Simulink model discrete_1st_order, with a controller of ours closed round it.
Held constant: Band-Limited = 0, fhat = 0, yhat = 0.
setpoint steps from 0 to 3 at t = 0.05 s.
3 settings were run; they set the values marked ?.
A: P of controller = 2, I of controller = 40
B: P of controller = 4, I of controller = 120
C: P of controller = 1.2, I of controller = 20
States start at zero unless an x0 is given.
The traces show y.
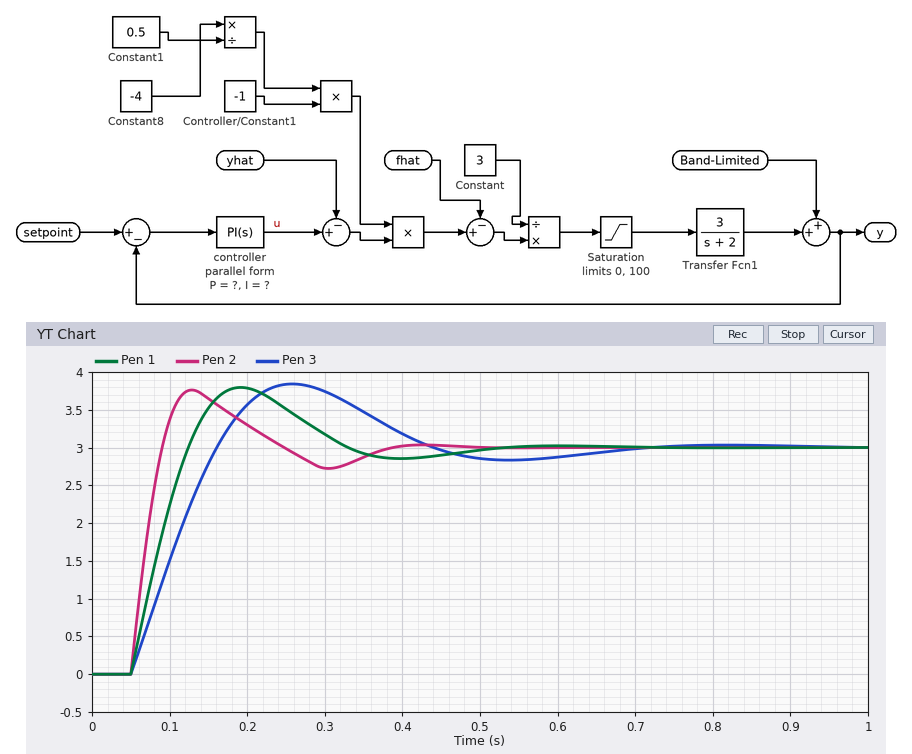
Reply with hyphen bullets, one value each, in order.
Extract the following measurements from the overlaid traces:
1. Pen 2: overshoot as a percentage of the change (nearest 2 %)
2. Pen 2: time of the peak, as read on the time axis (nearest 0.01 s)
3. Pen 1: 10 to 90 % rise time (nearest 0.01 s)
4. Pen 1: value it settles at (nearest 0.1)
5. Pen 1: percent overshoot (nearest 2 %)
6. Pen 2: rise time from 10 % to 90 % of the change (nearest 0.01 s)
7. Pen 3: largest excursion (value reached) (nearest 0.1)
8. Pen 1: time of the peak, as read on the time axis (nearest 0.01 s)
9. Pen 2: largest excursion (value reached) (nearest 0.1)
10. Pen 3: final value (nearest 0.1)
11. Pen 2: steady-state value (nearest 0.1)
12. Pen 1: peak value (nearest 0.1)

- 26 %
- 0.13 s
- 0.06 s
- 3.0
- 26 %
- 0.03 s
- 3.8
- 0.19 s
- 3.8
- 3.0
- 3.0
- 3.8
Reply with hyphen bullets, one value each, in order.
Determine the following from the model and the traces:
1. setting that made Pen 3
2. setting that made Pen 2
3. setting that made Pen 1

- C
- B
- A
